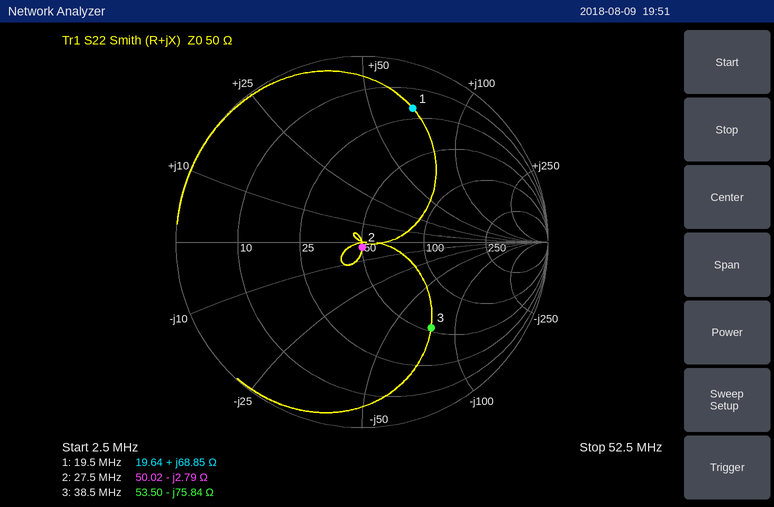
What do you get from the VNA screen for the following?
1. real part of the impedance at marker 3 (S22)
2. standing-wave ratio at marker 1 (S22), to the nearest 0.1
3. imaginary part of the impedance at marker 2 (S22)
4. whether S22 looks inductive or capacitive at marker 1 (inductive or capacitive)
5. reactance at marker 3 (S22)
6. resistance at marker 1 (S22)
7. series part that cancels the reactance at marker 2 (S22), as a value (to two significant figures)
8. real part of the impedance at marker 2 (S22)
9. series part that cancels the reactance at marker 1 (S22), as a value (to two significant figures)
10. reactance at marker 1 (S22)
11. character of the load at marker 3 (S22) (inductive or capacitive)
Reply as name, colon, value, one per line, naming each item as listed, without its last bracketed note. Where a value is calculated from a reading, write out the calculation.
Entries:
real part of the impedance at marker 3: 53.50 Ω
standing-wave ratio at marker 1 (S22), to the nearest 0.1: 7.6
imaginary part of the impedance at marker 2: -2.79 Ω
whether S22 looks inductive or capacitive at marker 1: inductive
reactance at marker 3: -75.84 Ω
resistance at marker 1: 19.64 Ω
series part that cancels the reactance at marker 2 (S22), as a value: L = 2.79 Ω/(2π × 27.5 MHz) ≈ 16 nH
real part of the impedance at marker 2: 50.02 Ω
series part that cancels the reactance at marker 1 (S22), as a value: C = 1/(2π × 19.5 MHz × 68.85 Ω) ≈ 119 pF, so 120 pF to two significant figures
reactance at marker 1: +68.85 Ω
character of the load at marker 3 (S22): capacitive
